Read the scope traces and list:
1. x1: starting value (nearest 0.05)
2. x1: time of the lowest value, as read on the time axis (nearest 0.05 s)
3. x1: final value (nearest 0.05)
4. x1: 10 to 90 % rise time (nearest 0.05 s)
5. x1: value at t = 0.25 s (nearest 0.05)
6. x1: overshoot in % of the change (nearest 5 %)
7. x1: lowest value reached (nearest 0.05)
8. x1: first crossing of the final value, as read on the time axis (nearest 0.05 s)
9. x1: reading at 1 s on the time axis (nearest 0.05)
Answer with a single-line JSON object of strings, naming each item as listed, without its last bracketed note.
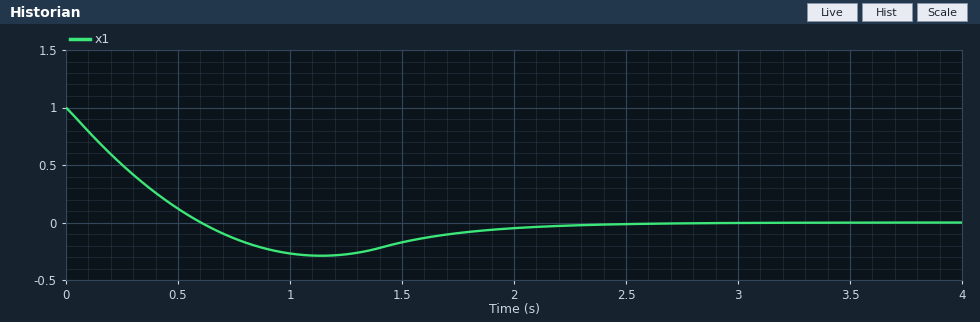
{"x1: starting value": "1.00", "x1: time of the lowest value, as read on the time axis": "1.15 s", "x1: final value": "0.00", "x1: 10 to 90 % rise time": "0.45 s", "x1: value at t = 0.25 s": "0.50", "x1: overshoot in % of the change": "30 %", "x1: lowest value reached": "-0.30", "x1: first crossing of the final value, as read on the time axis": "0.60 s", "x1: reading at 1 s on the time axis": "-0.25"}
